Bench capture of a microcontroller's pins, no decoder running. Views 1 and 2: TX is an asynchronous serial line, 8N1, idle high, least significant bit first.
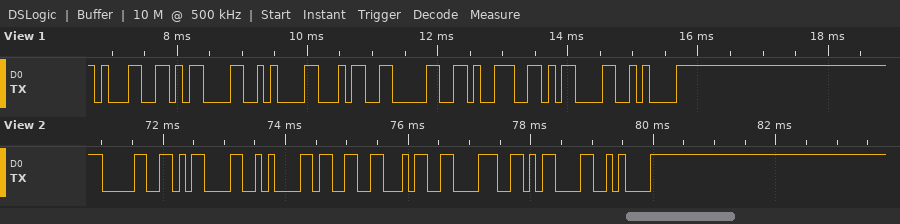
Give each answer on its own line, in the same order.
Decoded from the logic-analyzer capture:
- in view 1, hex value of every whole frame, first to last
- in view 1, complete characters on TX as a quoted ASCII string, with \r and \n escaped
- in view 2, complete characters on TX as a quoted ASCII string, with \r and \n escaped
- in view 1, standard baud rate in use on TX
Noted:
0x31 0x0D 0x0A 0x34 0x30 0x39 0x0D 0x0A
"1\r\n409\r\n"
"0\r\n348\r\n"
9600 baud
